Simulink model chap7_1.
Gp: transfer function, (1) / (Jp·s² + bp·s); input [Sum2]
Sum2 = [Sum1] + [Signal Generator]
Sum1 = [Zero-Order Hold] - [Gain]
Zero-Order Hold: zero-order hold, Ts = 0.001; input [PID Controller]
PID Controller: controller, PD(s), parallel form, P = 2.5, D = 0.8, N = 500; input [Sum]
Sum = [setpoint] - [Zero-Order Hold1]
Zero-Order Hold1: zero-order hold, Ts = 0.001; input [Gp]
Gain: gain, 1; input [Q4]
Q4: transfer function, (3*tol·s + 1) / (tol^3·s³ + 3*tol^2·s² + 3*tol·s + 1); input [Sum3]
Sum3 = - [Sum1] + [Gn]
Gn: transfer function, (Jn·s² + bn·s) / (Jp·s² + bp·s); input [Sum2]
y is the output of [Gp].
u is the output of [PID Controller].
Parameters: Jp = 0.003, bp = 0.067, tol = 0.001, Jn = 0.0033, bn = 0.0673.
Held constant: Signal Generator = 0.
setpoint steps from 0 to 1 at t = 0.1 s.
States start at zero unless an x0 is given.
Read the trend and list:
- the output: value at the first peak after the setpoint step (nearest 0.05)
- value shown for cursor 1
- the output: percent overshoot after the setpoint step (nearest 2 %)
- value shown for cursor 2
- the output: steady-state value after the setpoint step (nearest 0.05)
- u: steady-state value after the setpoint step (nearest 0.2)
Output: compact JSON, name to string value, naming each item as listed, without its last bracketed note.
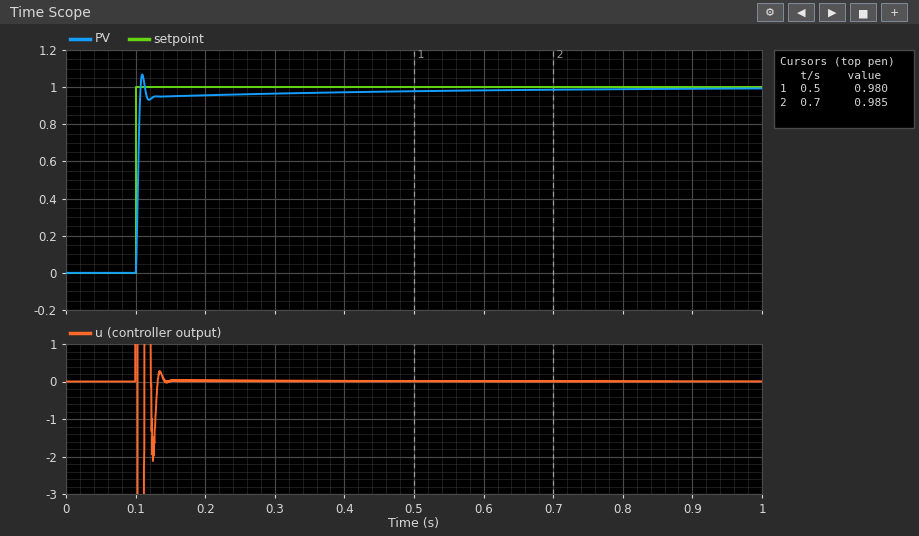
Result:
{"the output: value at the first peak after the setpoint step": "1.05", "value shown for cursor 1": "0.980", "the output: percent overshoot after the setpoint step": "6 %", "value shown for cursor 2": "0.985", "the output: steady-state value after the setpoint step": "1.00", "u: steady-state value after the setpoint step": "0.0"}
